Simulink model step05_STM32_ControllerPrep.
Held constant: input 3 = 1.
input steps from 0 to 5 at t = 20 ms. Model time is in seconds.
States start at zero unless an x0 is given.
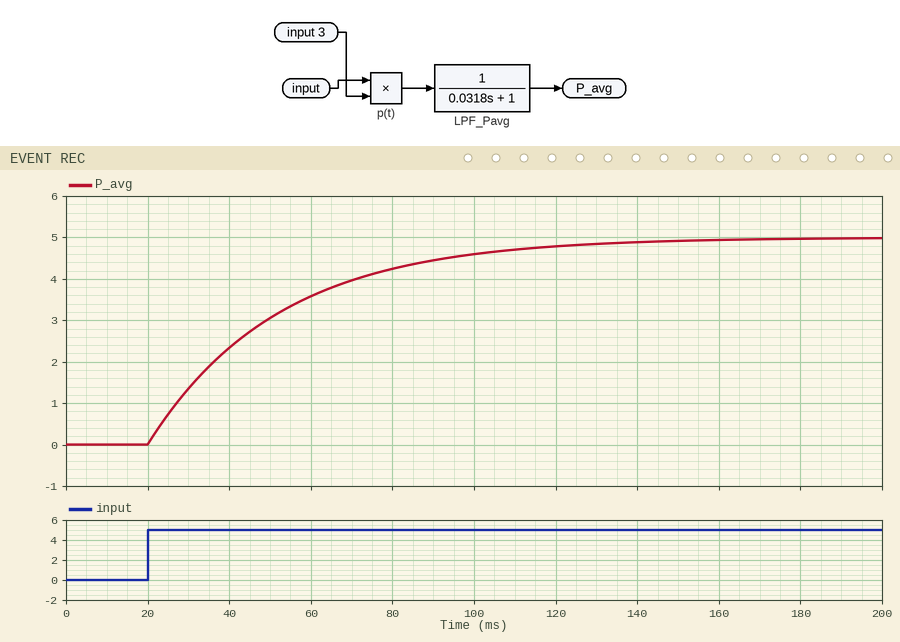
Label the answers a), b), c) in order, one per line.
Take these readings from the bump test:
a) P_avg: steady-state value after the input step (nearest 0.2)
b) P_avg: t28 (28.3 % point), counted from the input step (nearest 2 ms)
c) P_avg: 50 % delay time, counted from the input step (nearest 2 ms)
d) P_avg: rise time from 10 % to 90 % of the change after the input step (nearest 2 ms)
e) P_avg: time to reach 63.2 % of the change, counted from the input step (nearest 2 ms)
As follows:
a) 5.0
b) 10 ms
c) 22 ms
d) 70 ms
e) 32 ms
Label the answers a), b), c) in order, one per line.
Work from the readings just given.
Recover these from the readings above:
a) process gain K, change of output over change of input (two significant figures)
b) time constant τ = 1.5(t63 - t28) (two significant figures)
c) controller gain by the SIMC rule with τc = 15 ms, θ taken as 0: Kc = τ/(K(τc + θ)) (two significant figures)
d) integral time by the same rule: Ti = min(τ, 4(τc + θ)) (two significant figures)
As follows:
a) 1.0
b) 33 ms
c) 2.2
d) 33 ms
